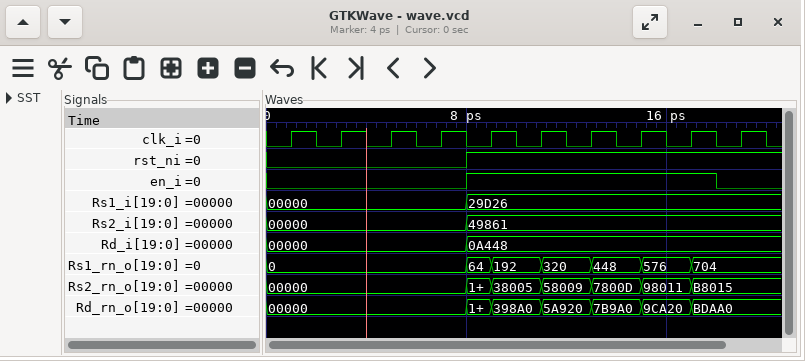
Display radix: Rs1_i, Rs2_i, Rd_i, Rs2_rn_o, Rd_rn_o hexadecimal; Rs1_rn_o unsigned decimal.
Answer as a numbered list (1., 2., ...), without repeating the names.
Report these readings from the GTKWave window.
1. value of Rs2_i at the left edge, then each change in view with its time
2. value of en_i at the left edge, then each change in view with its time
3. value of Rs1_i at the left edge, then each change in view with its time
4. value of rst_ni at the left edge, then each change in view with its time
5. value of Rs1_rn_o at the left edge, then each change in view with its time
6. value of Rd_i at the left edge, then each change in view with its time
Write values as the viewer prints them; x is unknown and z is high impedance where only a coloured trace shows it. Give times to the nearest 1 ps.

1. 00000, 49861 at 8 ps
2. 0, 1 at 8 ps, 0 at 18 ps
3. 00000, 29D26 at 8 ps
4. 0, 1 at 8 ps
5. 0, 64 at 8 ps, 192 at 9 ps, 320 at 11 ps, 448 at 13 ps, 576 at 15 ps, 704 at 17 ps
6. 00000, 0A448 at 8 ps
